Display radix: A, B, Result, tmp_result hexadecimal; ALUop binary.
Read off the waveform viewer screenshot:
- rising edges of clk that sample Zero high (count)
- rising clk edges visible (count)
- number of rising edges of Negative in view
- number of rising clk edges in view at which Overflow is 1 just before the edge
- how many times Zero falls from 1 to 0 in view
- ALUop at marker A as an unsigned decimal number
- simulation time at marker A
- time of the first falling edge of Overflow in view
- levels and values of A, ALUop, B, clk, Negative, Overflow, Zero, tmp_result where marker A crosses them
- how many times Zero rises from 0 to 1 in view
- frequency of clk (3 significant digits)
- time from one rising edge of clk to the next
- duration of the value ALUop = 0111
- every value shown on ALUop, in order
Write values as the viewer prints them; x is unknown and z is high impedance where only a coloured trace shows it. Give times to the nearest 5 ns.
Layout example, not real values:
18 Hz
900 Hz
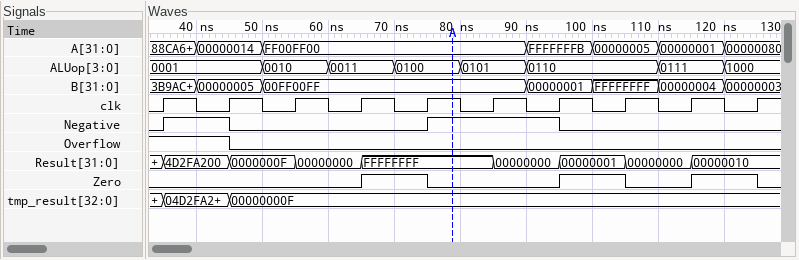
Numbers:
3
10
2
2
3
4
80 ns
45 ns
A=FF00FF00, ALUop=0100, B=00FF00FF, clk=1, Negative=1, Overflow=0, Zero=0, tmp_result=00000000F
3
100 MHz
10 ns
10 ns
0001, 0010, 0011, 0100, 0101, 0110, 0111, 1000
